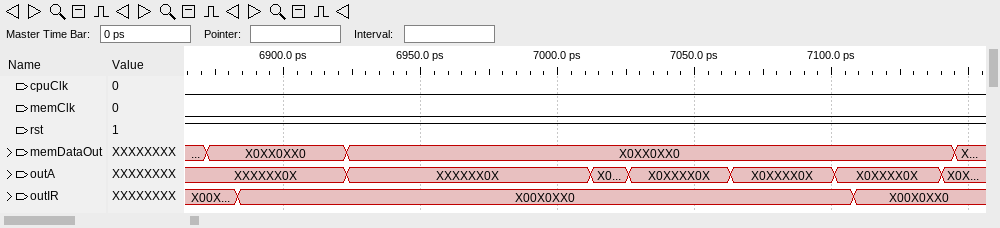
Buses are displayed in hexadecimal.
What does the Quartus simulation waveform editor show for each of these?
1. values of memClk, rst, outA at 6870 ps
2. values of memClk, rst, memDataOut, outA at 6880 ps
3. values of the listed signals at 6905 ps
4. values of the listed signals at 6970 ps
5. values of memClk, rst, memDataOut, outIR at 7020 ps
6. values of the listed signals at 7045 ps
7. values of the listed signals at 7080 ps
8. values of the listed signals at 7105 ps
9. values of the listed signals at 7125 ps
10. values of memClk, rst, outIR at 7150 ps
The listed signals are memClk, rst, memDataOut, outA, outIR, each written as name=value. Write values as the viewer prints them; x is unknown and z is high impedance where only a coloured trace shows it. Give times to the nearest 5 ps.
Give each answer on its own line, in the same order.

memClk=0, rst=1, outA=XXXXXX0X
memClk=0, rst=1, memDataOut=X0XX0XX0, outA=XXXXXX0X
memClk=0, rst=1, memDataOut=X0XX0XX0, outA=XXXXXX0X, outIR=X00X0XX0
memClk=0, rst=1, memDataOut=X0XX0XX0, outA=XXXXXX0X, outIR=X00X0XX0
memClk=0, rst=1, memDataOut=X0XX0XX0, outIR=X00X0XX0
memClk=0, rst=1, memDataOut=X0XX0XX0, outA=X0XXXX0X, outIR=X00X0XX0
memClk=0, rst=1, memDataOut=X0XX0XX0, outA=X0XXXX0X, outIR=X00X0XX0
memClk=0, rst=1, memDataOut=X0XX0XX0, outA=X0XXXX0X, outIR=X00X0XX0
memClk=0, rst=1, memDataOut=X0XX0XX0, outA=X0XXXX0X, outIR=X00X0XX0
memClk=0, rst=1, outIR=X00X0XX0
